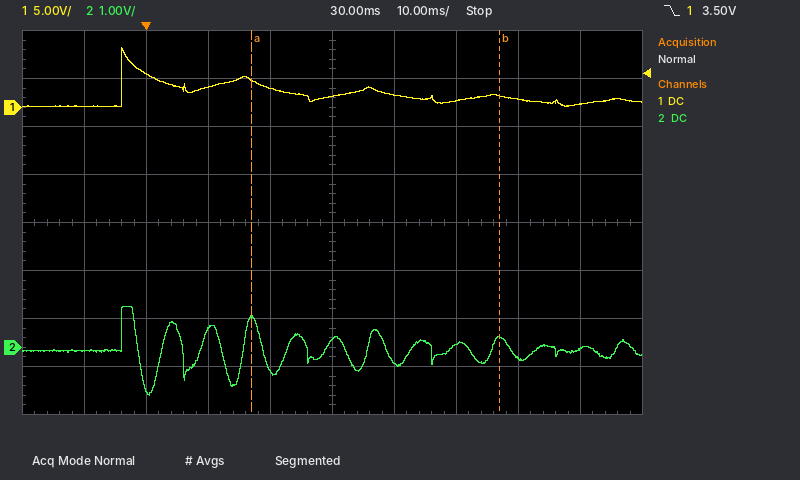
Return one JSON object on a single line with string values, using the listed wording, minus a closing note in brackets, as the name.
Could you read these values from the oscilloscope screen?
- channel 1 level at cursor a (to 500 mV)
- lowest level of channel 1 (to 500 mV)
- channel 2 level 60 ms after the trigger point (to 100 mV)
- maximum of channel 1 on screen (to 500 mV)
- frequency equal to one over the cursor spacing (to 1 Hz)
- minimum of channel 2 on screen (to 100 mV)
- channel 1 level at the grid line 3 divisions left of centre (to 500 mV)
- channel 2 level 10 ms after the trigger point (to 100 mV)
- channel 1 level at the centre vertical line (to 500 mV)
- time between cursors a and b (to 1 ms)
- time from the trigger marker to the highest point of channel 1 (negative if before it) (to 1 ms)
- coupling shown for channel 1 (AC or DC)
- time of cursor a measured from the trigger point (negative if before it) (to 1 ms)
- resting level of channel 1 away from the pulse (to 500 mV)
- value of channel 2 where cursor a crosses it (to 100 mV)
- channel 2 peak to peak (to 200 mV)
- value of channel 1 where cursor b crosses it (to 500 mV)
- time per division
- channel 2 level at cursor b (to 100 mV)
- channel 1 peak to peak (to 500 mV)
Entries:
{"channel 1 level at cursor a": "3.0 V", "lowest level of channel 1": "0.0 V", "channel 2 level 60 ms after the trigger point": "-200 mV", "maximum of channel 1 on screen": "6.0 V", "frequency equal to one over the cursor spacing": "25 Hz", "minimum of channel 2 on screen": "-1.0 V", "channel 1 level at the grid line 3 divisions left of centre": "3.5 V", "channel 2 level 10 ms after the trigger point": "400 mV", "channel 1 level at the centre vertical line": "1.0 V", "time between cursors a and b": "40 ms", "time from the trigger marker to the highest point of channel 1 (negative if before it)": "-4 ms", "coupling shown for channel 1": "DC", "time of cursor a measured from the trigger point (negative if before it)": "+17 ms", "resting level of channel 1 away from the pulse": "1.0 V", "value of channel 2 where cursor a crosses it": "600 mV", "channel 2 peak to peak": "1.8 V", "value of channel 1 where cursor b crosses it": "1.0 V", "time per division": "10 ms", "channel 2 level at cursor b": "200 mV", "channel 1 peak to peak": "6.0 V"}
